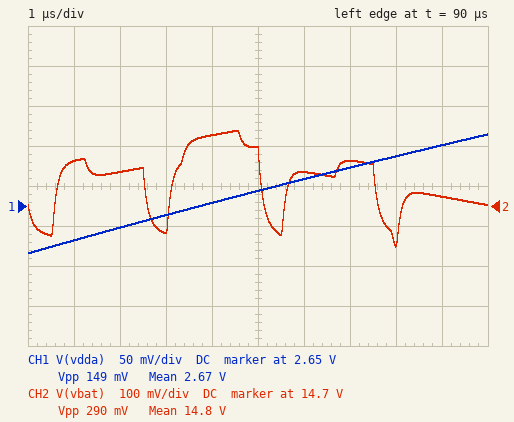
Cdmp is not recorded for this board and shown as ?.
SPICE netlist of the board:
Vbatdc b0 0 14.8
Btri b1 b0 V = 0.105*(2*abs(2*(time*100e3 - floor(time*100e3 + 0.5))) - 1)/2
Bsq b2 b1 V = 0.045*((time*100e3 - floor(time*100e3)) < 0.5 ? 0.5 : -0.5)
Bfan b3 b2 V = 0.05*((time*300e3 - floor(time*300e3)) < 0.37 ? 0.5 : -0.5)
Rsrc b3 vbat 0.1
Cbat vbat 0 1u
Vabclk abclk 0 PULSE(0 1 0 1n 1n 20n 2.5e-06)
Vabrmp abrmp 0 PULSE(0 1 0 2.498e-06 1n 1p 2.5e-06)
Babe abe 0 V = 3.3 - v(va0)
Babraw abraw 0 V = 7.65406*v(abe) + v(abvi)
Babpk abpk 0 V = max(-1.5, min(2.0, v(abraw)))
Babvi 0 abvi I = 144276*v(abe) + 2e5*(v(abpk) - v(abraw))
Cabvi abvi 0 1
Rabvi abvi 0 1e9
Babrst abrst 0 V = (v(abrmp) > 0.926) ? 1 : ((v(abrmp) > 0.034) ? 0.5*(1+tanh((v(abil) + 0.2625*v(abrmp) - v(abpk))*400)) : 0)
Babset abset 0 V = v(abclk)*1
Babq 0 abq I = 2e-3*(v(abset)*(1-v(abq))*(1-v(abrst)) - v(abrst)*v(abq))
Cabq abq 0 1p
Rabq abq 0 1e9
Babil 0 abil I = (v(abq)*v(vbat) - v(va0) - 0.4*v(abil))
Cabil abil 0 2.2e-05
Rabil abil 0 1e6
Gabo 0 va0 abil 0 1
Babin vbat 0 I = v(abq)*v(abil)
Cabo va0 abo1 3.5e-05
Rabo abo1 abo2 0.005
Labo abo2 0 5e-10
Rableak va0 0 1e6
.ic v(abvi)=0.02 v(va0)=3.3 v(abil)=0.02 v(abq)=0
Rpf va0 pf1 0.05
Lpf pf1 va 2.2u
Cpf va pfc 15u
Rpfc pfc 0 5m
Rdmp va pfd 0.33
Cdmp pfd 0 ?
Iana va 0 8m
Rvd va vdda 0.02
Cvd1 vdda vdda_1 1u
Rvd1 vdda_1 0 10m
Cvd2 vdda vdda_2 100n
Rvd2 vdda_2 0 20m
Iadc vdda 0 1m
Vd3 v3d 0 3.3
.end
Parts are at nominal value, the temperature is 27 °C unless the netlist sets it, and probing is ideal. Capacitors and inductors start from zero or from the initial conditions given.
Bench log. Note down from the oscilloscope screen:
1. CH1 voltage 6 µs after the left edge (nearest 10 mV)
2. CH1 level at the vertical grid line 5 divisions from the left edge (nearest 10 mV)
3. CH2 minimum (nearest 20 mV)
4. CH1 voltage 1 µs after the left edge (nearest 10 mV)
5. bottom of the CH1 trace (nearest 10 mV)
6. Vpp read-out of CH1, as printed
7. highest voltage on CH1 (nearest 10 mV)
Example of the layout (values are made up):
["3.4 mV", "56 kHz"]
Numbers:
["2.68 V", "2.67 V", "14.60 V", "2.61 V", "2.59 V", "149 mV", "2.74 V"]
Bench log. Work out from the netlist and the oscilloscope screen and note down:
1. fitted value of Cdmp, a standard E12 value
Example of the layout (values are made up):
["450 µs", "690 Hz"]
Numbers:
["56 µF"]
